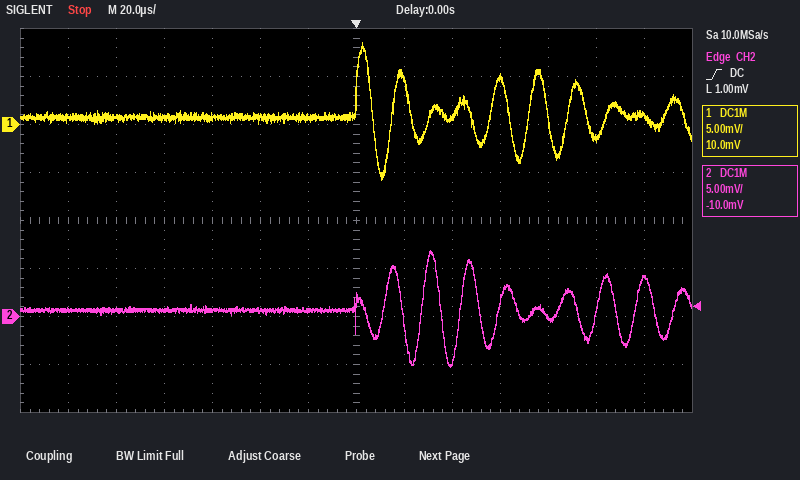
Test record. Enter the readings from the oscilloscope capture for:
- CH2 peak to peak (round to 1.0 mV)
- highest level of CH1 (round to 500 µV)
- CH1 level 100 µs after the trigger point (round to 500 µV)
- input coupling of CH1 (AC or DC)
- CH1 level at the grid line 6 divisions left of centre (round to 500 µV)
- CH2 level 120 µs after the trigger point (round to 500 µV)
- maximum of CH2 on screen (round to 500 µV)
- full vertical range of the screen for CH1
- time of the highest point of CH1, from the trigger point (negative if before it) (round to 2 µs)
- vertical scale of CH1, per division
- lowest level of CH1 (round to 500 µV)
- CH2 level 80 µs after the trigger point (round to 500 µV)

12.0 mV
8.5 mV
-1.5 mV
DC
500 µV
4.0 mV
7.0 mV
40 mV
+2 µs
5 mV
-5.5 mV
0.0 mV
